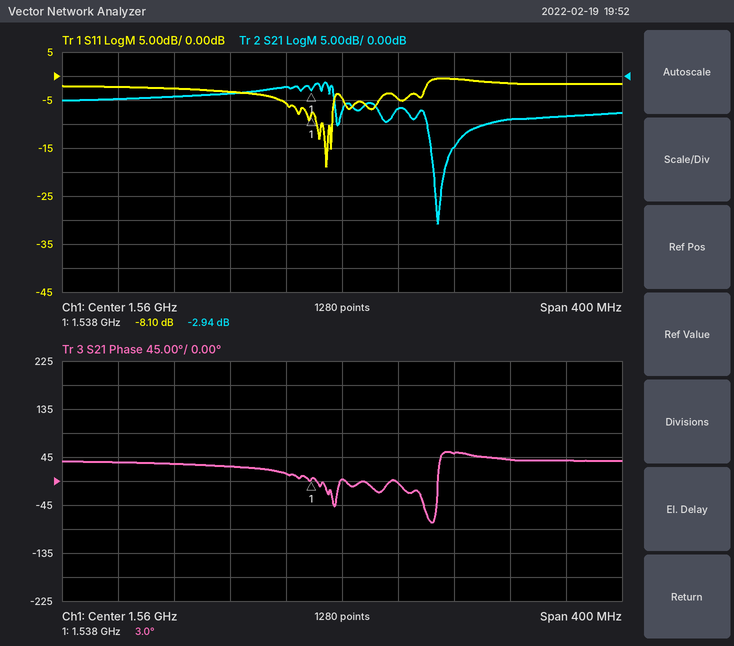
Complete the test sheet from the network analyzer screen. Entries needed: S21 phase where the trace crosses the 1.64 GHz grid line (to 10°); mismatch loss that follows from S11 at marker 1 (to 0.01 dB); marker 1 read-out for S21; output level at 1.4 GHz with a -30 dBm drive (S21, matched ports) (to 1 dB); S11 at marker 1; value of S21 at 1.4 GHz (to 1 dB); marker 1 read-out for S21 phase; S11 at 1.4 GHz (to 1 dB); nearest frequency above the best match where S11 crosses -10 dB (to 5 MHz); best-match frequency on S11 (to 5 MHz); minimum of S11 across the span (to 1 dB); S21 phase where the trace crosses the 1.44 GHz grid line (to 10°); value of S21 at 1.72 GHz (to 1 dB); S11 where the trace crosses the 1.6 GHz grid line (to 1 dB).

50°
0.73 dB
-2.94 dB
-35 dBm
-8.10 dB
-5 dB
3.0°
-2 dB
1.555 GHz
1.550 GHz
-19 dB
30°
-8 dB
-5 dB
